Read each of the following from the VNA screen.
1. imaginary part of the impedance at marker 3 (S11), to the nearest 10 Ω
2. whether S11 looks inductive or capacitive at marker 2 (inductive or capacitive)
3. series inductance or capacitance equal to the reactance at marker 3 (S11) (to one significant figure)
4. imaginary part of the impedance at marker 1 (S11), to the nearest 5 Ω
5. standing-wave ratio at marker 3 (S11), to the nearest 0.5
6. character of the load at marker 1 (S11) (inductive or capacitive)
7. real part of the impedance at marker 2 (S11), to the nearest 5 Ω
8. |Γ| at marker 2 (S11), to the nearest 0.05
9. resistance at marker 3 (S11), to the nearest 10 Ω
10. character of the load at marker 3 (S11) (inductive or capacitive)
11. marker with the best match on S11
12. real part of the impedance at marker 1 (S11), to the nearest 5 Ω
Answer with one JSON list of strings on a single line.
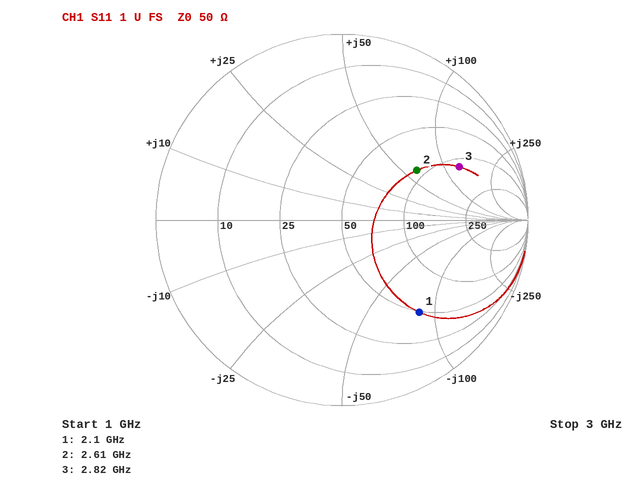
["+130 Ω", "inductive", "7 nH", "-85 Ω", "5.5", "capacitive", "90 Ω", "0.50", "120 Ω", "inductive", "marker 2", "50 Ω"]
